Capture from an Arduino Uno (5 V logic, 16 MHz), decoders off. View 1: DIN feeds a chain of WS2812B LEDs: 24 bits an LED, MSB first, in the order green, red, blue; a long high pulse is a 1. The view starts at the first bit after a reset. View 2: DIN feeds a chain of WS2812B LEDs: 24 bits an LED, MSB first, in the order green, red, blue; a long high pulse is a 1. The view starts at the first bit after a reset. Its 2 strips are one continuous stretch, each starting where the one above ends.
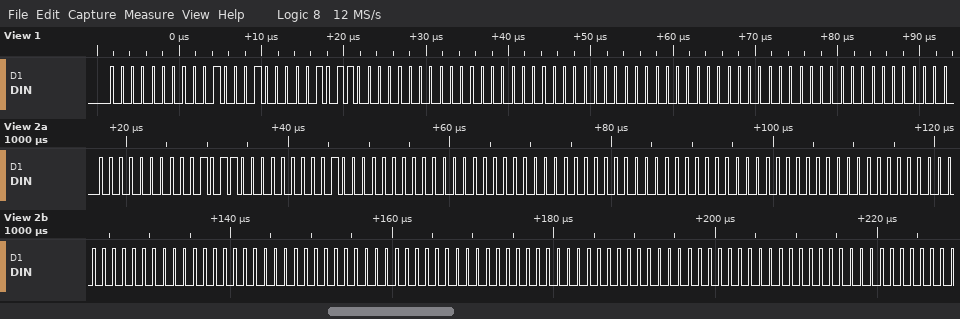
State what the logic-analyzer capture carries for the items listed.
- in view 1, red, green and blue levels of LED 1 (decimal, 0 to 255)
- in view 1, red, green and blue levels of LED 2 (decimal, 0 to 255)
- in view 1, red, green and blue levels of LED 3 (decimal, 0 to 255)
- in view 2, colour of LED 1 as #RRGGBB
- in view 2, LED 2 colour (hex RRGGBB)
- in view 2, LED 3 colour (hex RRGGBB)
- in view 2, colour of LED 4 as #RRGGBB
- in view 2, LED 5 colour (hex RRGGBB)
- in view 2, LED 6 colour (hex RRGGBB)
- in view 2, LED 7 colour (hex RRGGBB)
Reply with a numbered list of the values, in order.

1. 34, 0, 11
2. 0, 0, 0
3. 0, 0, 0
4. #2C0001
5. #000000
6. #000000
7. #000000
8. #000000
9. #000000
10. #000000
